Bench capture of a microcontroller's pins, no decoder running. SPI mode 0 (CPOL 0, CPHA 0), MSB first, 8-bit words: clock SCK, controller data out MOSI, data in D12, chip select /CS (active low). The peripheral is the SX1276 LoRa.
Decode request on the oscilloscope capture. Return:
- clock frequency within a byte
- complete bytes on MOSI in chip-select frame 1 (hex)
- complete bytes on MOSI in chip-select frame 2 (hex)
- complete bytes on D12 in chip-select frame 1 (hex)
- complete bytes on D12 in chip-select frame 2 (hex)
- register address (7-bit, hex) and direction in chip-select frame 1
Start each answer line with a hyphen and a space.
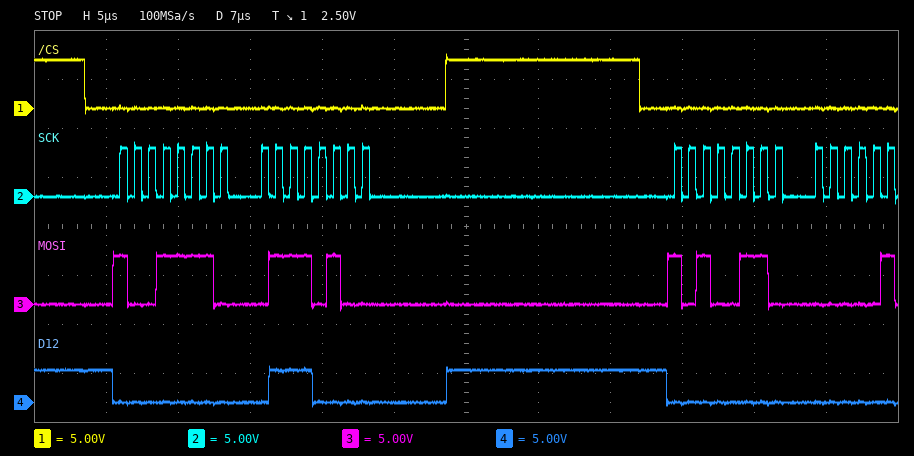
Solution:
- 1 MHz
- 9E 74
- A6
- 00 70
- 00
- 0x1E write
